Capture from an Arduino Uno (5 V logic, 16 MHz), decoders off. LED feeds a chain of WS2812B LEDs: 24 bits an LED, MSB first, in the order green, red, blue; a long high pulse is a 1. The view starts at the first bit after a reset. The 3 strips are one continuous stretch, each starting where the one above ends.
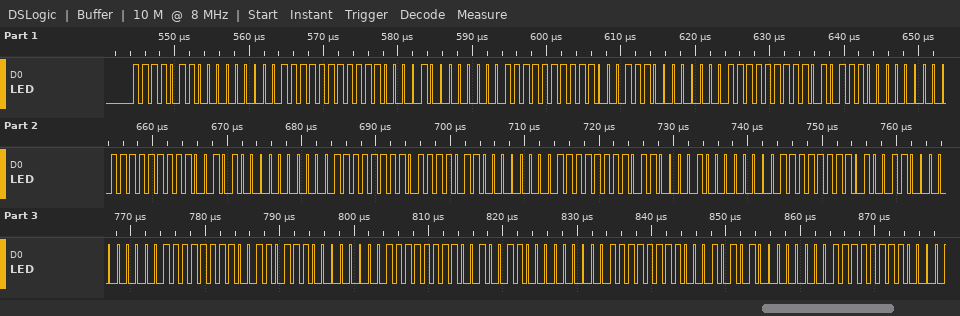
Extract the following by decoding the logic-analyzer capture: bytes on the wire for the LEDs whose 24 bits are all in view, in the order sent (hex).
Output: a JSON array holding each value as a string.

["F6 00 FF E1 00 FF C7 00 FF AE 00 FF 94 00 FF 7B 00 FF 61 00 FF 4C 00 FF 37 00 FF 26 00 FF 15 00 FF"]
